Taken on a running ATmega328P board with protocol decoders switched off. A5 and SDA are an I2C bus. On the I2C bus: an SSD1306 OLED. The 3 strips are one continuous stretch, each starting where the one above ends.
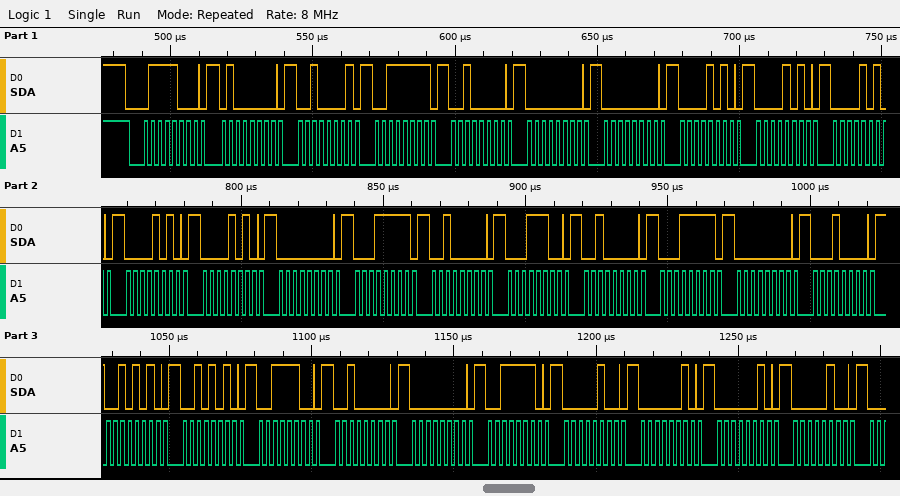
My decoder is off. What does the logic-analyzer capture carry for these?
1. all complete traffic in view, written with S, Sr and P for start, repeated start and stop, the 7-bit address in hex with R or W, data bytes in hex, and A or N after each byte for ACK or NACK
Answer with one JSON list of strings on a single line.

["S 3CW A 40 A 21 A 3F A 20 A 00 A 00 A 0A A 0A A 0A A 0A A 0A A 00 A 1F A 20 A 1C A 20 A 1F A 00 A 10 A 2A A 2A A 3C A 20 A 00 A 3E A 04 A 02 A 02 A 04 A"]
